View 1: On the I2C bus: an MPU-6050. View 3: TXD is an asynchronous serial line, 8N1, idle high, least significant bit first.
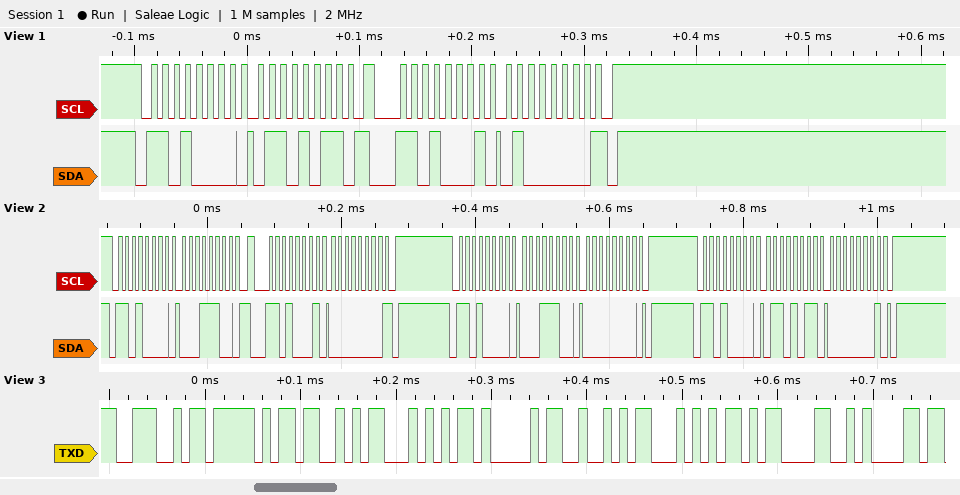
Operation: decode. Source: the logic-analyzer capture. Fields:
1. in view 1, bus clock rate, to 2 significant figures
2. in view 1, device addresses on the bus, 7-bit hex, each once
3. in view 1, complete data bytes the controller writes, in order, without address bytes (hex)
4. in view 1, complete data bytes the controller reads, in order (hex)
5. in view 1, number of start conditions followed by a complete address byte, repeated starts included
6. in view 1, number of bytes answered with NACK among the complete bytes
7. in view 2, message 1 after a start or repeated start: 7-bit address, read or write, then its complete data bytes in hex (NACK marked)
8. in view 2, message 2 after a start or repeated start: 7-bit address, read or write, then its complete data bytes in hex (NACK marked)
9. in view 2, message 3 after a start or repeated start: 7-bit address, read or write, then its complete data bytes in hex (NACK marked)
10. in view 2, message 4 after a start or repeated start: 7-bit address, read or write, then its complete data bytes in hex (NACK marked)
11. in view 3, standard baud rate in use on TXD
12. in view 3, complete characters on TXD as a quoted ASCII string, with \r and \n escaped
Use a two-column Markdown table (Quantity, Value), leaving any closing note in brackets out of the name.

| Quantity | Value |
|---|---|
| in view 1, bus clock rate, to 2 significant figures | 100 kHz |
| in view 1, device addresses on the bus, 7-bit hex, each once | 0x68 |
| in view 1, complete data bytes the controller writes, in order, without address bytes | 6B |
| in view 1, complete data bytes the controller reads, in order | 40 |
| in view 1, number of start conditions followed by a complete address byte, repeated starts included | 2 |
| in view 1, number of bytes answered with NACK among the complete bytes | 1 |
| in view 2, message 1 after a start or repeated start: 7-bit address, read or write, then its complete data bytes in hex | 0x68 write: 1C |
| in view 2, message 2 after a start or repeated start: 7-bit address, read or write, then its complete data bytes in hex | 0x68 read: 00 NACK |
| in view 2, message 3 after a start or repeated start: 7-bit address, read or write, then its complete data bytes in hex | 0x68 write: 1C 00 |
| in view 2, message 4 after a start or repeated start: 7-bit address, read or write, then its complete data bytes in hex | 0x68 write: 6B 01 |
| in view 3, standard baud rate in use on TXD | 115200 baud |
| in view 3, complete characters on TXD as a quoted ASCII string, with \r and \n escaped | "N_START\r\n" |
